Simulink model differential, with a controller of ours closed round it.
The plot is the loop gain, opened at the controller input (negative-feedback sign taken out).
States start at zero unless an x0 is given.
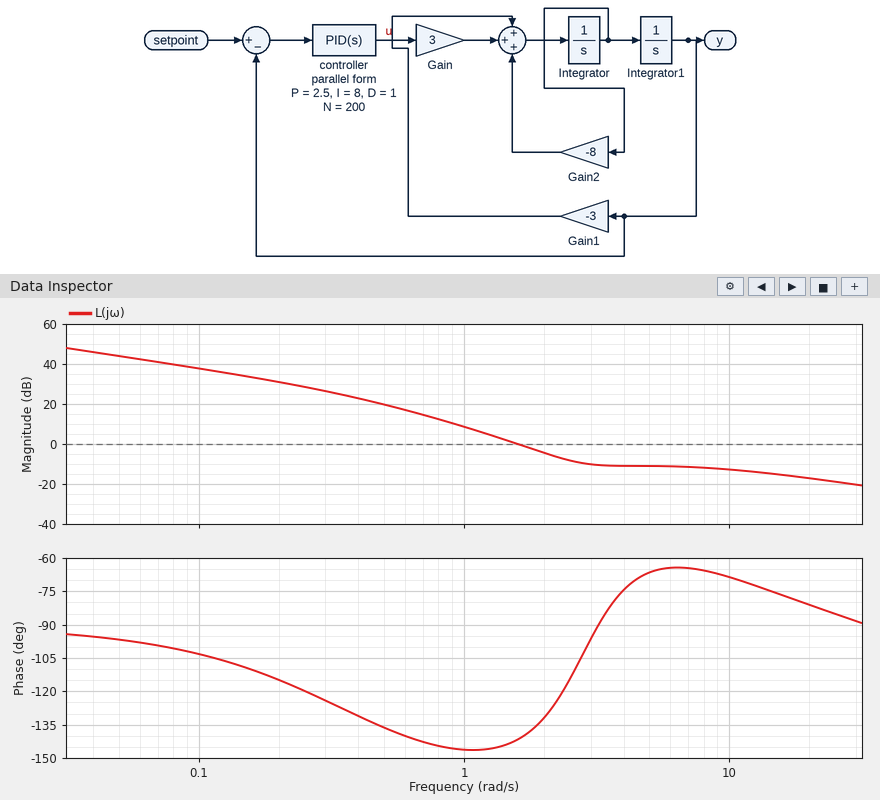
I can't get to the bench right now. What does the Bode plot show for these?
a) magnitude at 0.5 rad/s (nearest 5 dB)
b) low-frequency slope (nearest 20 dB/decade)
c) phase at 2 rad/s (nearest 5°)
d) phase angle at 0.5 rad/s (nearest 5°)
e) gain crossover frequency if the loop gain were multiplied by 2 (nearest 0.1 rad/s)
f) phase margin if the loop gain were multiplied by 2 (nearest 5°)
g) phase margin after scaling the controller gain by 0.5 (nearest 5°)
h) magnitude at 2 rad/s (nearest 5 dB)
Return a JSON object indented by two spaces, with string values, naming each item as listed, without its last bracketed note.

{
  "magnitude at 0.5 rad/s": "20 dB",
  "low-frequency slope": "-20 dB/decade",
  "phase at 2 rad/s": "-130°",
  "phase angle at 0.5 rad/s": "-135°",
  "gain crossover frequency if the loop gain were multiplied by 2": "2.2 rad/s",
  "phase margin if the loop gain were multiplied by 2": "55°",
  "phase margin after scaling the controller gain by 0.5": "35°",
  "magnitude at 2 rad/s": "-5 dB"
}
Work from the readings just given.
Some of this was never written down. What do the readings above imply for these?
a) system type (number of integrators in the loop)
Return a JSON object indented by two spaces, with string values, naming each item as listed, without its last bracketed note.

{
  "system type": "1"
}
